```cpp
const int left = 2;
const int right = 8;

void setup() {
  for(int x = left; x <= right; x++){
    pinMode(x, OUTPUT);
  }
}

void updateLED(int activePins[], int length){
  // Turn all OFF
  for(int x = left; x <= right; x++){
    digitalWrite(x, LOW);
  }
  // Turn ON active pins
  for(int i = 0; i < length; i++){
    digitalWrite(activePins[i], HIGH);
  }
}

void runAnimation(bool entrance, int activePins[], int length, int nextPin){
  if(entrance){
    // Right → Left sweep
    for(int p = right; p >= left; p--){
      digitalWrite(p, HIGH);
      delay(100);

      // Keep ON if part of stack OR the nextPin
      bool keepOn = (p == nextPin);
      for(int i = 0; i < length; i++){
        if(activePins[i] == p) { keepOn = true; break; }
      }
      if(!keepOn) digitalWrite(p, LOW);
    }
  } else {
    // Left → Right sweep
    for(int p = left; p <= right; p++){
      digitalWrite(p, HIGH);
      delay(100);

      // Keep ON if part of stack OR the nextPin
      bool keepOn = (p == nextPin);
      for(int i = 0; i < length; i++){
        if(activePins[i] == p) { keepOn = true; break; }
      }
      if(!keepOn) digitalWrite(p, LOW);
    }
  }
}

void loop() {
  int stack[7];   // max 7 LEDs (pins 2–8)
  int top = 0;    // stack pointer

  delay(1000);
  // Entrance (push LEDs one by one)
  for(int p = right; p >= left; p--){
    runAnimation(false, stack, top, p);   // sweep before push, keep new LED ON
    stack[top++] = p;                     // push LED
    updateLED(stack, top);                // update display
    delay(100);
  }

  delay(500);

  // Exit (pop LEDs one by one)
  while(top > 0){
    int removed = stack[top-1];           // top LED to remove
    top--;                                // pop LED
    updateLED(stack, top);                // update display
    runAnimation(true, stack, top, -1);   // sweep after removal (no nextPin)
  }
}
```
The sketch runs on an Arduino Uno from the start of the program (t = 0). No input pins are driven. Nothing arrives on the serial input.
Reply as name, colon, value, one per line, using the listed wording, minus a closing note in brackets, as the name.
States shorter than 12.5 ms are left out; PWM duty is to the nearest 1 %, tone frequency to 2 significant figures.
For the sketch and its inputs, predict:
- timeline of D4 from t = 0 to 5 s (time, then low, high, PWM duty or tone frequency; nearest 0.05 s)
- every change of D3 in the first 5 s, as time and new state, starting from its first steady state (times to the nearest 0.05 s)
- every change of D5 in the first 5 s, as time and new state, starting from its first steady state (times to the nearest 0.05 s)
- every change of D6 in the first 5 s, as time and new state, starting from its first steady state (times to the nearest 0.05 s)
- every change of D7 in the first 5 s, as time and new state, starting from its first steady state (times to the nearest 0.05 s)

timeline of D4 from t = 0 to 5 s: 0 s low; 1.2 s high; 1.3 s low; 2 s high; 2.1 s low; 2.8 s high; 2.9 s low; 3.6 s high; 3.7 s low; 4.4 s high
every change of D3 in the first 5 s, as time and new state, starting from its first steady state: 0 s low; 1.1 s high; 1.2 s low; 1.9 s high; 2 s low; 2.7 s high; 2.8 s low; 3.5 s high; 3.6 s low; 4.3 s high; 4.4 s low
every change of D5 in the first 5 s, as time and new state, starting from its first steady state: 0 s low; 1.3 s high; 1.4 s low; 2.1 s high; 2.2 s low; 2.9 s high; 3 s low; 3.7 s high
every change of D6 in the first 5 s, as time and new state, starting from its first steady state: 0 s low; 1.4 s high; 1.5 s low; 2.2 s high; 2.3 s low; 3 s high
every change of D7 in the first 5 s, as time and new state, starting from its first steady state: 0 s low; 1.5 s high; 1.6 s low; 2.3 s high
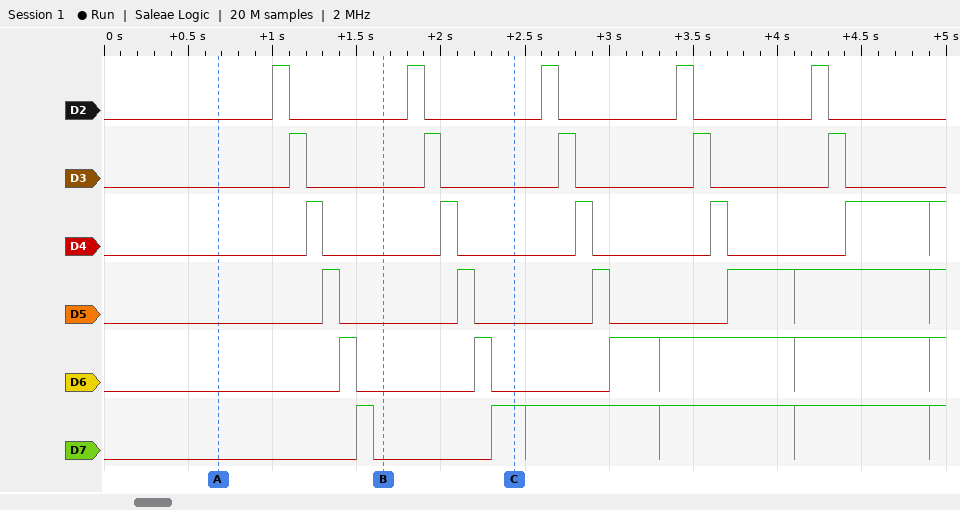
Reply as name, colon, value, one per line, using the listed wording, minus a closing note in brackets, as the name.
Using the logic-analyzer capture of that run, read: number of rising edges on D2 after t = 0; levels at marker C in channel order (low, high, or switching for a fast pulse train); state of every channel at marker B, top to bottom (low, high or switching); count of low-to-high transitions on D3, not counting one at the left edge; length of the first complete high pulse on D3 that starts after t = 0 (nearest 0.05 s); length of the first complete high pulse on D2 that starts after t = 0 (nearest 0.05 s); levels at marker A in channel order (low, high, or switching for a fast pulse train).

number of rising edges on D2 after t = 0: 5
levels at marker C in channel order: D2 low, D3 low, D4 low, D5 low, D6 low, D7 high
state of every channel at marker B, top to bottom: D2 low, D3 low, D4 low, D5 low, D6 low, D7 low
count of low-to-high transitions on D3, not counting one at the left edge: 5
length of the first complete high pulse on D3 that starts after t = 0: 0.10 s
length of the first complete high pulse on D2 that starts after t = 0: 0.10 s
levels at marker A in channel order: D2 low, D3 low, D4 low, D5 low, D6 low, D7 low
